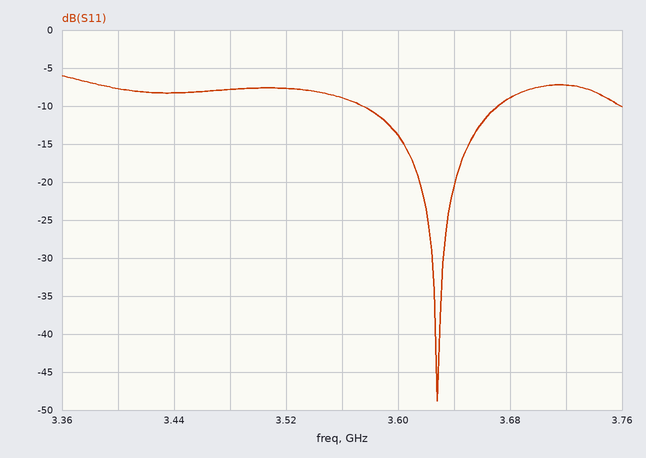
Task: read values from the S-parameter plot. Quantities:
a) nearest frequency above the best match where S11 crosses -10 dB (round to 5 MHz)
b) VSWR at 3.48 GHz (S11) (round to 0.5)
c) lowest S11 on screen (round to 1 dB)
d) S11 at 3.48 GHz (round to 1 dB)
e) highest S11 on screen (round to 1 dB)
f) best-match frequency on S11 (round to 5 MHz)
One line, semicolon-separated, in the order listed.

3.670 GHz; 2.5; -49 dB; -8 dB; -6 dB; 3.630 GHz
